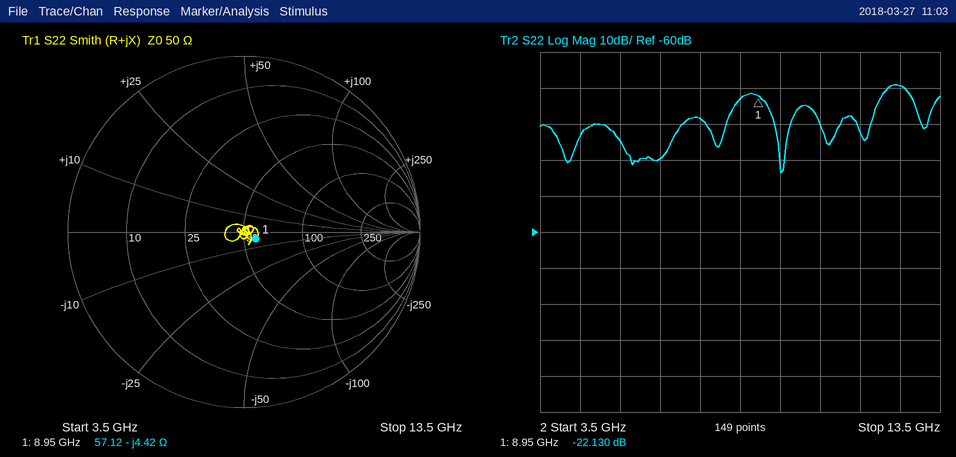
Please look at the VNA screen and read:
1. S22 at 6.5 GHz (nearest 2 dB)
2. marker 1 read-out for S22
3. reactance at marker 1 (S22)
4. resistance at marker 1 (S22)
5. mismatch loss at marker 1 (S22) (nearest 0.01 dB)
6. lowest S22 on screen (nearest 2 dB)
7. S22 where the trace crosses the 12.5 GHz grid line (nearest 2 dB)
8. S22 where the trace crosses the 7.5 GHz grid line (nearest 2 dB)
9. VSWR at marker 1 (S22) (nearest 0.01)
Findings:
-40 dB
-22.130 dB
-4.42 Ω
57.12 Ω
0.03 dB
-44 dB
-20 dB
-28 dB
1.17
